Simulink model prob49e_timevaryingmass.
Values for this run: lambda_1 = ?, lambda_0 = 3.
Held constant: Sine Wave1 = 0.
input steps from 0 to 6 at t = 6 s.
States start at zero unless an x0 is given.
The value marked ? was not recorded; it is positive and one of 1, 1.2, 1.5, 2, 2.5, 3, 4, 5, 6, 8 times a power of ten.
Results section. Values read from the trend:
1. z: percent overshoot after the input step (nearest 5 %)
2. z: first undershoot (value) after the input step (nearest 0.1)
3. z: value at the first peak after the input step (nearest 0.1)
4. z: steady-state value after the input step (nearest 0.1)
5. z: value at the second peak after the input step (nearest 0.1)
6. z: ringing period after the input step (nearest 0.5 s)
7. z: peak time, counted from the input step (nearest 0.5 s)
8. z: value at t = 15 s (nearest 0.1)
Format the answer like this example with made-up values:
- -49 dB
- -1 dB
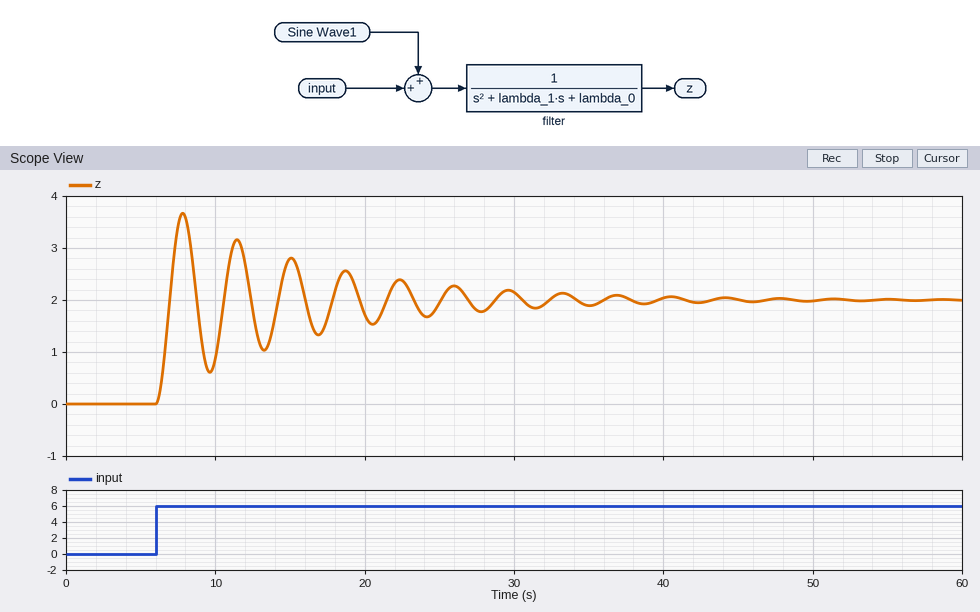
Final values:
- 85 %
- 0.6
- 3.7
- 2.0
- 3.2
- 3.5 s
- 2.0 s
- 2.8
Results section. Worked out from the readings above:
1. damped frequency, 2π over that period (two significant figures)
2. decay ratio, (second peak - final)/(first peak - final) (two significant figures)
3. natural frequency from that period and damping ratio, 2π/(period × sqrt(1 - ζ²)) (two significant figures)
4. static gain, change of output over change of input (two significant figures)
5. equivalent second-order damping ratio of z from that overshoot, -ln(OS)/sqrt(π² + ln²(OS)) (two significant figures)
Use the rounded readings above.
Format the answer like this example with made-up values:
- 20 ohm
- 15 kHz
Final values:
- 1.8 rad/s
- 0.71
- 1.8 rad/s
- 0.33
- 0.052
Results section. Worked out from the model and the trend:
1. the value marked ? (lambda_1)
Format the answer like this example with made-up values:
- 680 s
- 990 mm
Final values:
- 0.2
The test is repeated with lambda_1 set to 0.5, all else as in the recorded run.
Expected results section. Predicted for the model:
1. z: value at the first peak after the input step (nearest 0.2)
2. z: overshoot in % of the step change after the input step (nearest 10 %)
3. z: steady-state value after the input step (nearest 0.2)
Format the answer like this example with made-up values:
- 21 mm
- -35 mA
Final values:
- 3.2
- 60 %
- 2.0
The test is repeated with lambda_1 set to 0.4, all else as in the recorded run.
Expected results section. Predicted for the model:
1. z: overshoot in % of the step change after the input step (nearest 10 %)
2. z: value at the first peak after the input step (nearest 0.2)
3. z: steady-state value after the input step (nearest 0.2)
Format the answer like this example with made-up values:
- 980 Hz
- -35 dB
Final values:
- 70 %
- 3.4
- 2.0
